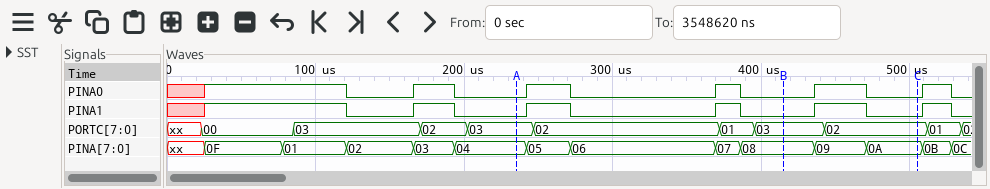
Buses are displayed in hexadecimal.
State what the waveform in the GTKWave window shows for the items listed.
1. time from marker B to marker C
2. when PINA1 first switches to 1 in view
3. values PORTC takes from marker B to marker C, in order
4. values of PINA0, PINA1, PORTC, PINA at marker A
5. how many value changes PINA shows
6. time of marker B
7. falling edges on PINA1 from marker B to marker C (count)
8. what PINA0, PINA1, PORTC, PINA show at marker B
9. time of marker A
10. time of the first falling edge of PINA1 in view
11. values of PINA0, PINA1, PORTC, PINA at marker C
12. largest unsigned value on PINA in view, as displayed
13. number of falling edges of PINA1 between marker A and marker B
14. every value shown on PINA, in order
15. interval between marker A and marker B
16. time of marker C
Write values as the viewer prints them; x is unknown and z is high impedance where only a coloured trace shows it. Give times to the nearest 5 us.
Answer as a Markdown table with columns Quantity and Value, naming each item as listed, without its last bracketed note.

| Quantity | Value |
|---|---|
| time from marker B to marker C | 90 us |
| when PINA1 first switches to 1 in view | 25 us |
| values PORTC takes from marker B to marker C, in order | 03, 02 |
| values of PINA0, PINA1, PORTC, PINA at marker A | PINA0=0, PINA1=0, PORTC=03, PINA=04 |
| how many value changes PINA shows | 13 |
| time of marker B | 415 us |
| falling edges on PINA1 from marker B to marker C | 1 |
| what PINA0, PINA1, PORTC, PINA show at marker B | PINA0=0, PINA1=0, PORTC=03, PINA=08 |
| time of marker A | 235 us |
| time of the first falling edge of PINA1 in view | 120 us |
| values of PINA0, PINA1, PORTC, PINA at marker C | PINA0=0, PINA1=0, PORTC=02, PINA=0A |
| largest unsigned value on PINA in view, as displayed | 0F |
| number of falling edges of PINA1 between marker A and marker B | 2 |
| every value shown on PINA, in order | xx, 0F, 01, 02, 03, 04, 05, 06, 07, 08, 09, 0A, 0B, 0C |
| interval between marker A and marker B | 180 us |
| time of marker C | 505 us |
